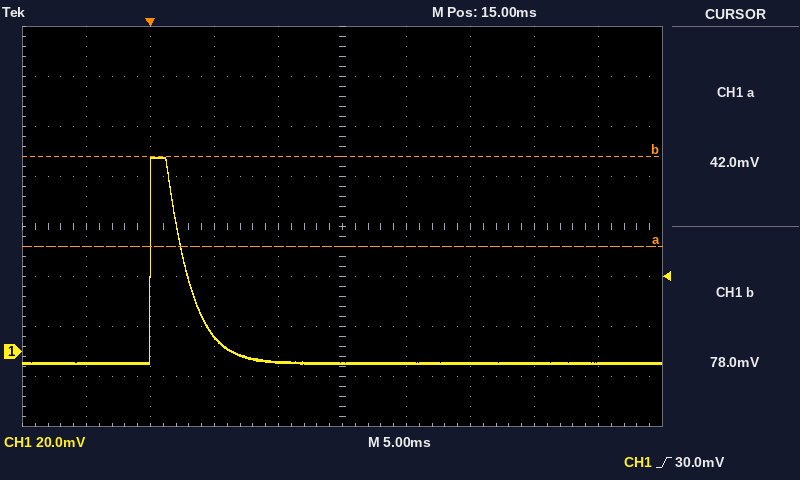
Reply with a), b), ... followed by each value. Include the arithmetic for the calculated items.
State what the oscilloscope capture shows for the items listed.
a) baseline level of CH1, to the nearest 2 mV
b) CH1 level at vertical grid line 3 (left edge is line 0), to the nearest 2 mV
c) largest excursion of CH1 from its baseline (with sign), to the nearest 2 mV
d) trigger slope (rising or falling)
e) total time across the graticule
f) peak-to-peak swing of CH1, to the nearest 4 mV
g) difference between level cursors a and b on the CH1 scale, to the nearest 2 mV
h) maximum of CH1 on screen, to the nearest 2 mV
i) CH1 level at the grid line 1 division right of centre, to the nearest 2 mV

a) -4 mV
b) 6 mV
c) 78 mV − (-4 mV) = +82 mV
d) rising
e) 50 ms
f) 84 mV
g) 36 mV
h) 78 mV
i) -4 mV
